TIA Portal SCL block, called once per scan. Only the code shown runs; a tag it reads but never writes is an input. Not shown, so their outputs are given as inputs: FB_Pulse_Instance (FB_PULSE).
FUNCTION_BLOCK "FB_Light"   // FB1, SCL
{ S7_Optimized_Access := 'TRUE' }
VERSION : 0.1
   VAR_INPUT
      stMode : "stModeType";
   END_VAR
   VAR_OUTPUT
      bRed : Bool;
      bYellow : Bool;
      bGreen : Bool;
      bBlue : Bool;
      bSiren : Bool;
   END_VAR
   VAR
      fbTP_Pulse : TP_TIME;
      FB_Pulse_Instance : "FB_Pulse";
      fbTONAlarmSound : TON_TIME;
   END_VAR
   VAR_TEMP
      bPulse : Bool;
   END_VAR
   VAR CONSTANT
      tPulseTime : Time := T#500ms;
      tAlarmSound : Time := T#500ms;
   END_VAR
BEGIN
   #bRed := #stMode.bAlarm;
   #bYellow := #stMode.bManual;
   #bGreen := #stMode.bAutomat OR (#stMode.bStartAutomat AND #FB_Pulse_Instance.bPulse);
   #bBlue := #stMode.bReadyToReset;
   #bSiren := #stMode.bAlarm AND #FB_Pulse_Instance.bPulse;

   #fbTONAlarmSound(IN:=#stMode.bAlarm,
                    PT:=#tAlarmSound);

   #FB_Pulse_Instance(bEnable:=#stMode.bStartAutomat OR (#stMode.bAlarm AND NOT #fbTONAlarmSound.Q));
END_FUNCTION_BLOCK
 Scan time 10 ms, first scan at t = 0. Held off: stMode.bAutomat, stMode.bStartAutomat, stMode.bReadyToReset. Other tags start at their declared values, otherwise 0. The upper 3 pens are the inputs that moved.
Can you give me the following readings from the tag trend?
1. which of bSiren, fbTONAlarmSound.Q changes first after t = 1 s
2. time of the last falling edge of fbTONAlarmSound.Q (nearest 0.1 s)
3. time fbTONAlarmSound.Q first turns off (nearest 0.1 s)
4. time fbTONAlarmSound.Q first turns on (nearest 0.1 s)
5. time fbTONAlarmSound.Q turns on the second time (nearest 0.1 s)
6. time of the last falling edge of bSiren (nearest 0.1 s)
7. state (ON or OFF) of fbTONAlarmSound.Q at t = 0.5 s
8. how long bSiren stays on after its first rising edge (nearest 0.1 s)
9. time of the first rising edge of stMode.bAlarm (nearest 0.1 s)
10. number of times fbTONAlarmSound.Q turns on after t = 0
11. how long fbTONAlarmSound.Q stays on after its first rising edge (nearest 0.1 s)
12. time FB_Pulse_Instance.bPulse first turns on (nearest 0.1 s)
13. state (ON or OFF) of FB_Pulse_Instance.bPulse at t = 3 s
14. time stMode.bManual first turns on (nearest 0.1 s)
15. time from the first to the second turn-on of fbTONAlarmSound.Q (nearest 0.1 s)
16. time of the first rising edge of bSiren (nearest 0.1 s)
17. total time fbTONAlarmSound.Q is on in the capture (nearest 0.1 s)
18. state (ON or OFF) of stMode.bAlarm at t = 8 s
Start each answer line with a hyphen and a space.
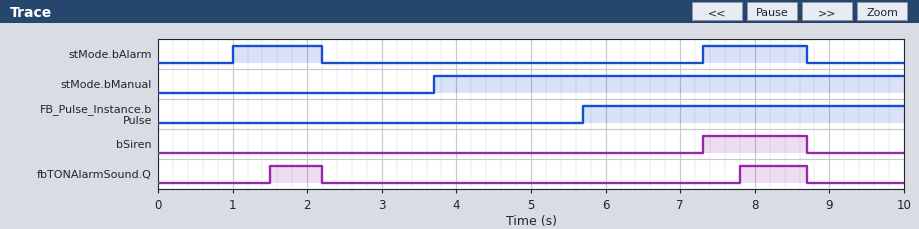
- fbTONAlarmSound.Q
- 8.7 s
- 2.2 s
- 1.5 s
- 7.8 s
- 8.7 s
- OFF
- 1.4 s
- 1.0 s
- 2
- 0.7 s
- 5.7 s
- OFF
- 3.7 s
- 6.3 s
- 7.3 s
- 1.6 s
- ON
